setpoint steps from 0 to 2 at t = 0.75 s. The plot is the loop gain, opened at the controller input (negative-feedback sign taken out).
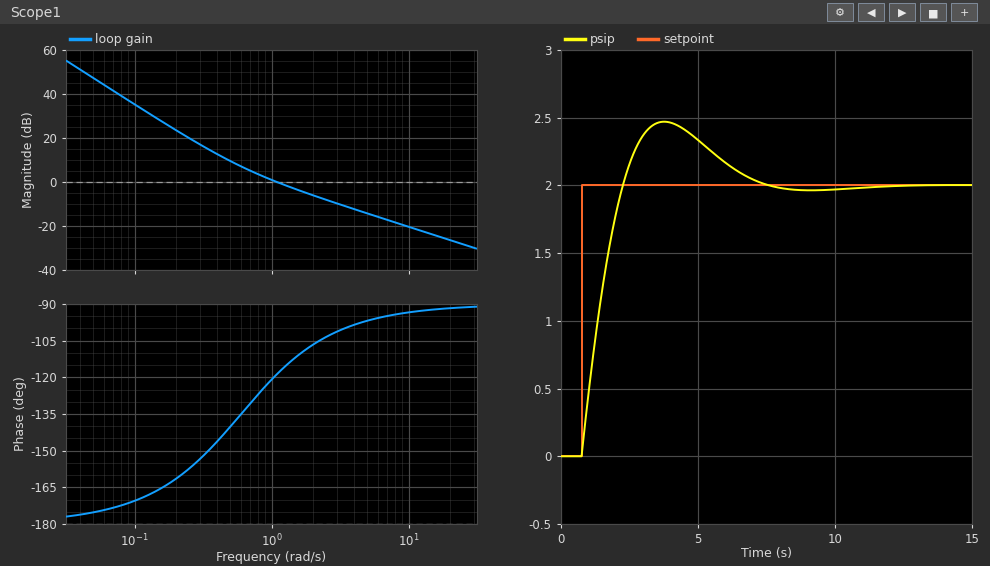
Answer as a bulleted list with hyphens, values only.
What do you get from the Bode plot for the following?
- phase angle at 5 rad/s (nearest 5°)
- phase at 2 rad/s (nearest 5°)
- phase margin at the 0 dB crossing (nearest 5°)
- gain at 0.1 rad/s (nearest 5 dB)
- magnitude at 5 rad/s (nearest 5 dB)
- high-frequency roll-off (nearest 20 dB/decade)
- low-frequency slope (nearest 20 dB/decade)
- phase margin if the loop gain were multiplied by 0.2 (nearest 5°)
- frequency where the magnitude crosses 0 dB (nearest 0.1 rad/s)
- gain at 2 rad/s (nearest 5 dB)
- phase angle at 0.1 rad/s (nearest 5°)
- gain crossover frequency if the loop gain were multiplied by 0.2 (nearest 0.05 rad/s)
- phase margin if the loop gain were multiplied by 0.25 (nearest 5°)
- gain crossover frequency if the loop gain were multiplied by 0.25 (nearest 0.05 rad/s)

- -95°
- -105°
- 60°
- 35 dB
- -15 dB
- -20 dB/decade
- -40 dB/decade
- 30°
- 1.1 rad/s
- -5 dB
- -170°
- 0.35 rad/s
- 35°
- 0.40 rad/s
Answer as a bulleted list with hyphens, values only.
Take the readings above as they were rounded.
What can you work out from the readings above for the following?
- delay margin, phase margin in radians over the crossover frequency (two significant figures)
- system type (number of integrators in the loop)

- 0.95 s
- 2
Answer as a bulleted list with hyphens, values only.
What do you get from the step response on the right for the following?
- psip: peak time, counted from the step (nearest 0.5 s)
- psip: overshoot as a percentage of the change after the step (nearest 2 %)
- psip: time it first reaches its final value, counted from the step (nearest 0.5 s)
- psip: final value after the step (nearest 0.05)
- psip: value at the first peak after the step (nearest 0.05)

- 3.0 s
- 24 %
- 1.5 s
- 2.00
- 2.45
